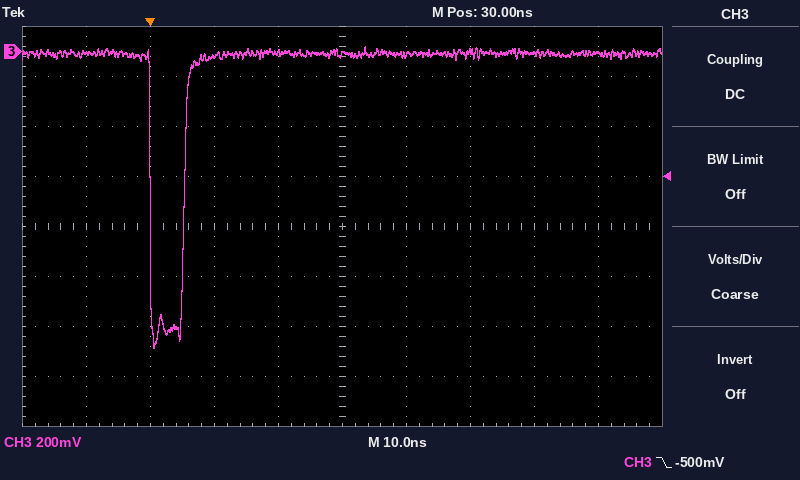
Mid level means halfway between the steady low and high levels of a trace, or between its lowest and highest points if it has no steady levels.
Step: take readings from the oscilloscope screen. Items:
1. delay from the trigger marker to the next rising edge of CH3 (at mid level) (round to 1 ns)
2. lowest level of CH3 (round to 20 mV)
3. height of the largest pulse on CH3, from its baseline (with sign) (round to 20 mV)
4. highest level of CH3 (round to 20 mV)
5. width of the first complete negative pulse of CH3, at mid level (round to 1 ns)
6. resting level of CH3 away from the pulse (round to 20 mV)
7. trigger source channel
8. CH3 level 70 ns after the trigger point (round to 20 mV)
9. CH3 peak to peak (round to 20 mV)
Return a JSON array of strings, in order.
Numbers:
["5 ns", "-1.18 V", "-1.18 V", "20 mV", "5 ns", "0 mV", "CH3", "0 mV", "1.20 V"]
